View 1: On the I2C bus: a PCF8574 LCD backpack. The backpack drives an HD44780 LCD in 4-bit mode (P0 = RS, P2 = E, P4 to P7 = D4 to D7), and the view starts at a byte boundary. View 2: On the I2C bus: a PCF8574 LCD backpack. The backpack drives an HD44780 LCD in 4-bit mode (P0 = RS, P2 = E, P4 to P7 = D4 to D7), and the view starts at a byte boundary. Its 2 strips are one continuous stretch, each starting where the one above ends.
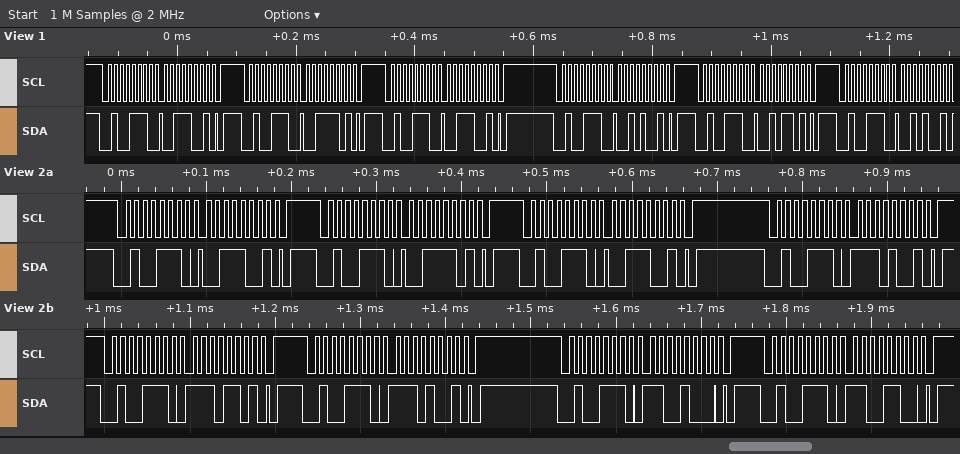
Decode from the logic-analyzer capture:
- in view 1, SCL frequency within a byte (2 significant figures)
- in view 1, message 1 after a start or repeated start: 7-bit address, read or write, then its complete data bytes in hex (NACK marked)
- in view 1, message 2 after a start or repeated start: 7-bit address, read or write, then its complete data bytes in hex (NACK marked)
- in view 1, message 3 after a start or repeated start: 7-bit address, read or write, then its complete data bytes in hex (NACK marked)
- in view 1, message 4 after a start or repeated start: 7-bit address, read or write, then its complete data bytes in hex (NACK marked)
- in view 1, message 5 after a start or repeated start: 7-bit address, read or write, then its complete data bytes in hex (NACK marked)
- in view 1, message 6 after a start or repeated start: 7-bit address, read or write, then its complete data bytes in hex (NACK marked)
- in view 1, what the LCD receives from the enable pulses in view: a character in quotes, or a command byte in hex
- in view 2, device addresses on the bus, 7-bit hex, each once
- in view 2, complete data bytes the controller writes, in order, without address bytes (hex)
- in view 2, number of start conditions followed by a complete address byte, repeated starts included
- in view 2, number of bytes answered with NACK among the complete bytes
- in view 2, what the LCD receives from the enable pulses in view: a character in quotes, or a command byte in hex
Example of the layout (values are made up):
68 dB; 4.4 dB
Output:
100 kHz; 0x27 write: 39; 0x27 write: 3D; 0x27 write: 39; 0x27 write: 29; 0x27 write: 2D; 0x27 write: 29; '2'; 0x27; 39 3D 39 E9 ED E9 C8 CC; 8; 0; '>'
